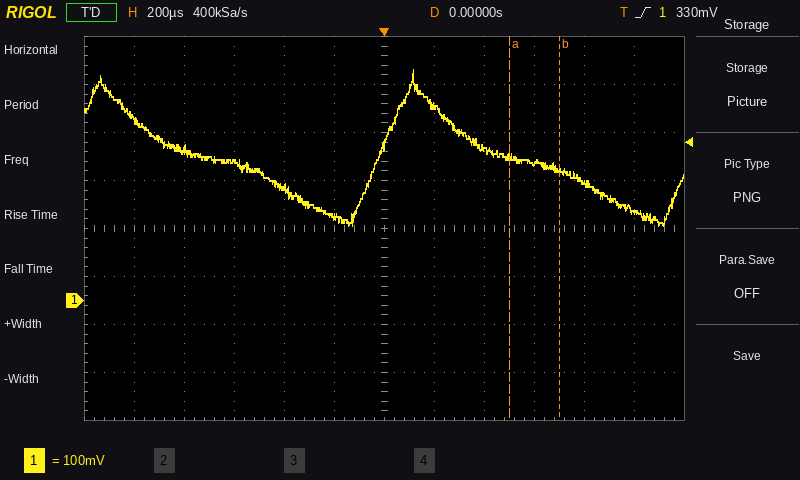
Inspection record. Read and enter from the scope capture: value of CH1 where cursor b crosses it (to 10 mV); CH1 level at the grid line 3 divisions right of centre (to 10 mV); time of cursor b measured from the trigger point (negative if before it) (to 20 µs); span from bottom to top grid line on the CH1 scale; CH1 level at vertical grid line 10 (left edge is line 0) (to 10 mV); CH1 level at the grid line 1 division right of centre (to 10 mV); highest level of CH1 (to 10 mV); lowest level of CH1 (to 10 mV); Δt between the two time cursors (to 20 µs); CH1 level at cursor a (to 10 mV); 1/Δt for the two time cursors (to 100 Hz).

270 mV
290 mV
+700 µs
800 mV
240 mV
410 mV
480 mV
160 mV
200 µs
300 mV
5.0 kHz
